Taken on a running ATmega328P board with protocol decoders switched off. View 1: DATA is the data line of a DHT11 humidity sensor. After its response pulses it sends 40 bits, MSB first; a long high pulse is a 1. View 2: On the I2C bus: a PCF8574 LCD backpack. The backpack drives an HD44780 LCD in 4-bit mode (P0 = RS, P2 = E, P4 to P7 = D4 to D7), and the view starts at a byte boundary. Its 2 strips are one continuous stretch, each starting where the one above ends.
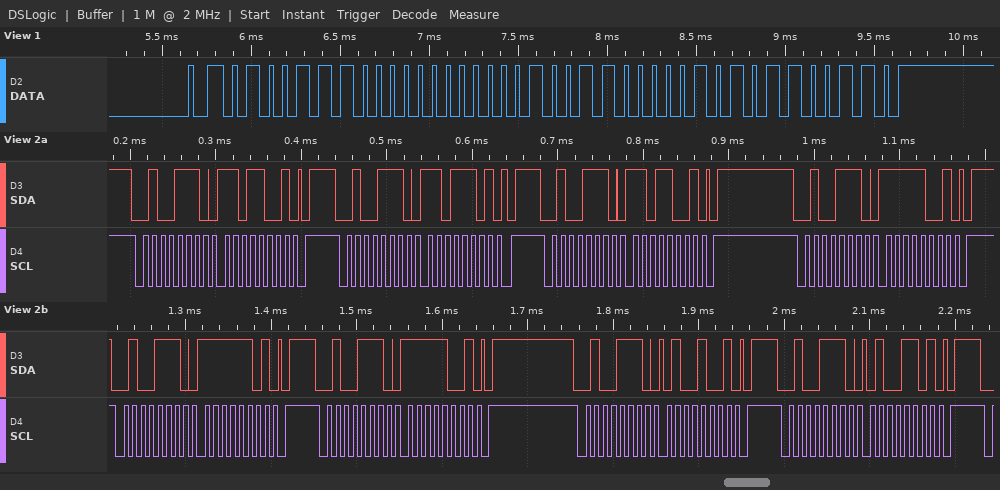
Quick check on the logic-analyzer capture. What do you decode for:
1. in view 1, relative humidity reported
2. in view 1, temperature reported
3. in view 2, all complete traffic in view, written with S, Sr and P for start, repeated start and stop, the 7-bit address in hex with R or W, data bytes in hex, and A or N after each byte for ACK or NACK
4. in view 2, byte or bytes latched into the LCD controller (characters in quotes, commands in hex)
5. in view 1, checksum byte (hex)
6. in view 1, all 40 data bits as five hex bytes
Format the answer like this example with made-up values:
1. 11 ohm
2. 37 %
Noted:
1. 78 %
2. 19.5 °C
3. S 27W A D9 A P S 27W A DD A P S 27W A D9 A P S 27W A F9 A P S 27W A FD A P S 27W A F9 A P S 27W A 49 A P S 27W A 4D A P
4. data 0xDF
5. 0x66
6. 4E 00 13 05 66
